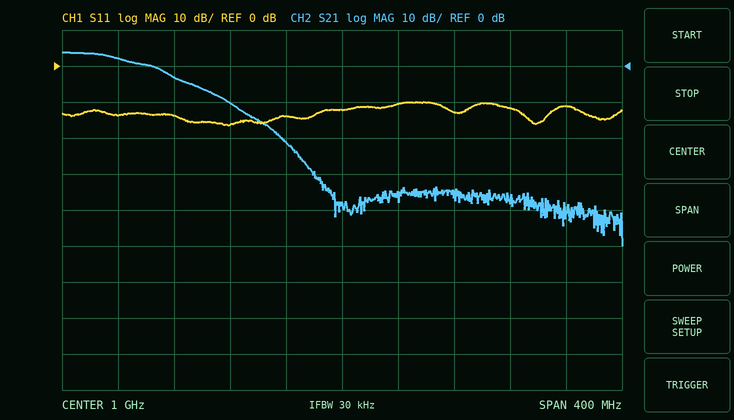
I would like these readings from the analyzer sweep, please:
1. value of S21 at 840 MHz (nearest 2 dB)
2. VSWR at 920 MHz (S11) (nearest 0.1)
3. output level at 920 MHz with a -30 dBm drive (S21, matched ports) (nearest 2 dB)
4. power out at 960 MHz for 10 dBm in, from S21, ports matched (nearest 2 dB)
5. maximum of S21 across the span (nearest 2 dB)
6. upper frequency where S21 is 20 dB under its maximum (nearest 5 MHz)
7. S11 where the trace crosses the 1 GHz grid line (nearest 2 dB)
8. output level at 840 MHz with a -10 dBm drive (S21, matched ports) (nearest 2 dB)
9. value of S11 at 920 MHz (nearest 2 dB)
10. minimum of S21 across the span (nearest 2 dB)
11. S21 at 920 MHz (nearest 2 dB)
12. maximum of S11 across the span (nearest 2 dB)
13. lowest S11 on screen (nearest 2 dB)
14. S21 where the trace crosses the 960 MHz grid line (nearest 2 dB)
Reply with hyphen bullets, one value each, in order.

- 2 dB
- 1.4
- -40 dBm
- -12 dBm
- 4 dB
- 945 MHz
- -12 dB
- -8 dBm
- -16 dB
- -50 dB
- -10 dB
- -10 dB
- -16 dB
- -22 dB
